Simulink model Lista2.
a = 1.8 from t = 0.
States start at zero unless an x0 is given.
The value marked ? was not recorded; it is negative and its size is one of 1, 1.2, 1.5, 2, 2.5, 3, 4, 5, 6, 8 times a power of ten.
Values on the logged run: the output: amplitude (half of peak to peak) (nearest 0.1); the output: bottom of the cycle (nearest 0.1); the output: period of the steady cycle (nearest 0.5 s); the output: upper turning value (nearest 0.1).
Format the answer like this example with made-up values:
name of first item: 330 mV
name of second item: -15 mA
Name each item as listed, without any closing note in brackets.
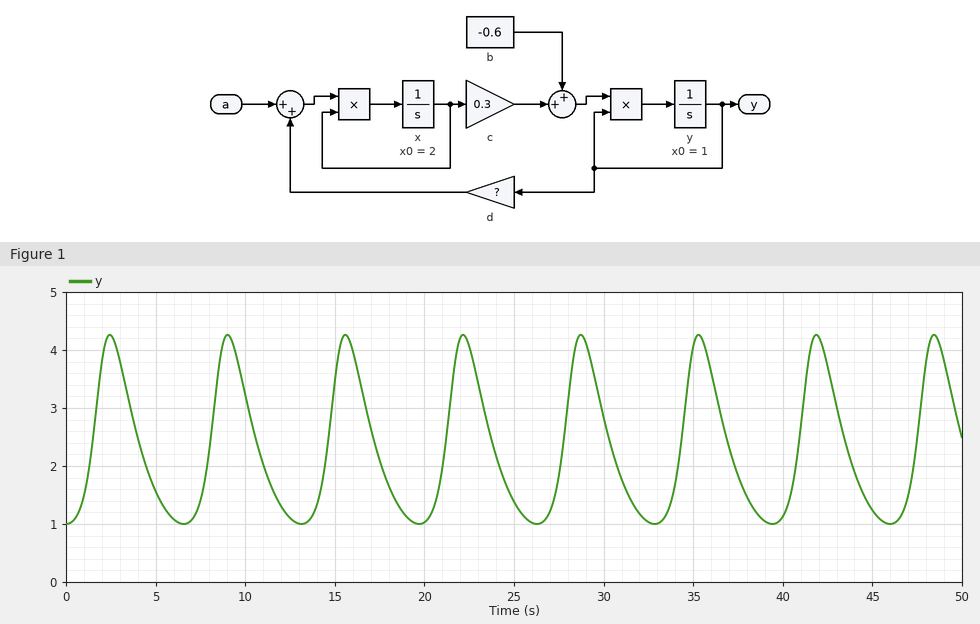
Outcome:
the output: amplitude (half of peak to peak): 1.6
the output: bottom of the cycle: 1.0
the output: period of the steady cycle: 6.5 s
the output: upper turning value: 4.3
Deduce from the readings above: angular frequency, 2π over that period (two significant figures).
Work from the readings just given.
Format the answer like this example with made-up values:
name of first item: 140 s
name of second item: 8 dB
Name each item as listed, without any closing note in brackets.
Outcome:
angular frequency, 2π over that period: 0.97 rad/s
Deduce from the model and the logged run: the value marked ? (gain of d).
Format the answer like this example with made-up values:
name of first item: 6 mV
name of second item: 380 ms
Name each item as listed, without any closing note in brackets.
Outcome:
the value marked ?: -0.8
